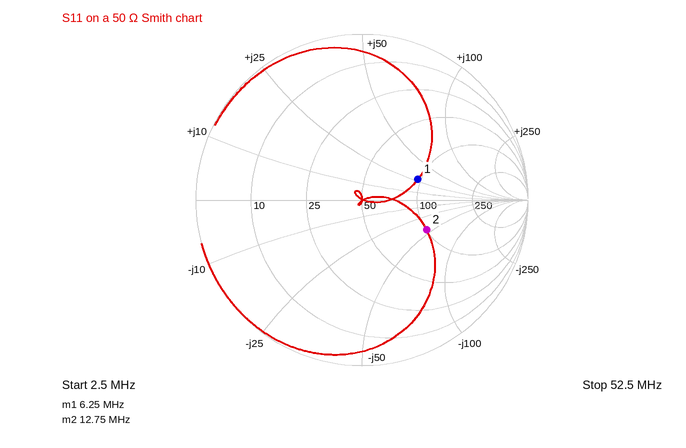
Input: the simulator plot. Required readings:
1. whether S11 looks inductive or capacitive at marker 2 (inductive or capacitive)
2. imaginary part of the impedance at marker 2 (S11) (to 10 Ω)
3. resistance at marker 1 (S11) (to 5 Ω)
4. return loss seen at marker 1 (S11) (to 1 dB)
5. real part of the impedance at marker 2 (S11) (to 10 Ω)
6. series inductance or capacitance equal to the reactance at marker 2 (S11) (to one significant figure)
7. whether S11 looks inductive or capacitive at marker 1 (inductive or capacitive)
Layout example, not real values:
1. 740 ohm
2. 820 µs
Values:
1. capacitive
2. -40 Ω
3. 95 Ω
4. 9 dB
5. 100 Ω
6. 300 pF
7. inductive
